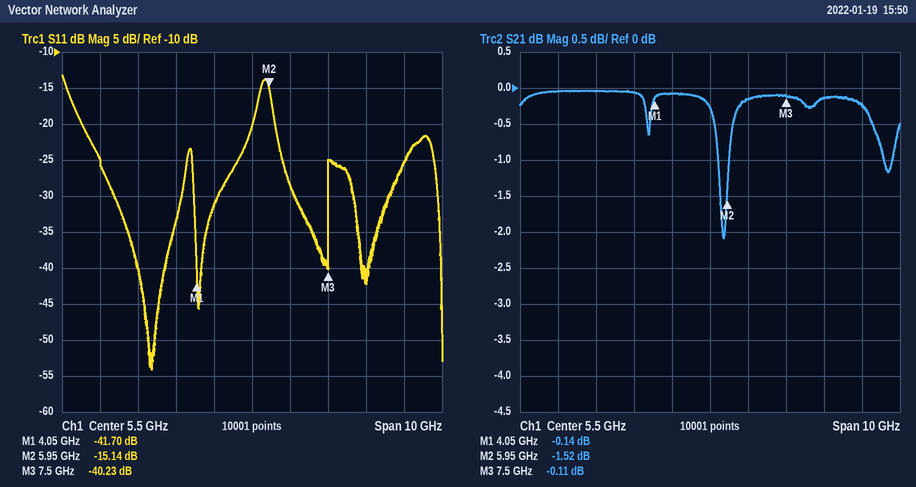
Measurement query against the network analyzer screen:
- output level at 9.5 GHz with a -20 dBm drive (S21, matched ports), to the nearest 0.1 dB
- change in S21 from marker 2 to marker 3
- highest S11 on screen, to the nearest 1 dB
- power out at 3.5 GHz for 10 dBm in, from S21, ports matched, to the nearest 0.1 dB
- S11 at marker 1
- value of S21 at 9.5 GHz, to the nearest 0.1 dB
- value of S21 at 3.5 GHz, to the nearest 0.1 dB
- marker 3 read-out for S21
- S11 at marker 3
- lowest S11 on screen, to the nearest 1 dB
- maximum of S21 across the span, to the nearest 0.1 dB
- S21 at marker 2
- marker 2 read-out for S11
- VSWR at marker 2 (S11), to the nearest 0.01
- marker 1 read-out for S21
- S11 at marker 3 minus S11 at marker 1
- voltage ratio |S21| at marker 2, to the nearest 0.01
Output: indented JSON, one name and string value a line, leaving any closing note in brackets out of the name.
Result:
{
  "output level at 9.5 GHz with a -20 dBm drive (S21, matched ports), to the nearest 0.1 dB": "-20.2 dBm",
  "change in S21 from marker 2 to marker 3": "1.41 dB",
  "highest S11 on screen, to the nearest 1 dB": "-13 dB",
  "power out at 3.5 GHz for 10 dBm in, from S21, ports matched, to the nearest 0.1 dB": "9.9 dBm",
  "S11 at marker 1": "-41.70 dB",
  "value of S21 at 9.5 GHz, to the nearest 0.1 dB": "-0.2 dB",
  "value of S21 at 3.5 GHz, to the nearest 0.1 dB": "-0.1 dB",
  "marker 3 read-out for S21": "-0.11 dB",
  "S11 at marker 3": "-40.23 dB",
  "lowest S11 on screen, to the nearest 1 dB": "-54 dB",
  "maximum of S21 across the span, to the nearest 0.1 dB": "0.0 dB",
  "S21 at marker 2": "-1.52 dB",
  "marker 2 read-out for S11": "-15.14 dB",
  "VSWR at marker 2 (S11), to the nearest 0.01": "1.42",
  "marker 1 read-out for S21": "-0.14 dB",
  "S11 at marker 3 minus S11 at marker 1": "1.47 dB",
  "voltage ratio |S21| at marker 2, to the nearest 0.01": "0.84"
}
